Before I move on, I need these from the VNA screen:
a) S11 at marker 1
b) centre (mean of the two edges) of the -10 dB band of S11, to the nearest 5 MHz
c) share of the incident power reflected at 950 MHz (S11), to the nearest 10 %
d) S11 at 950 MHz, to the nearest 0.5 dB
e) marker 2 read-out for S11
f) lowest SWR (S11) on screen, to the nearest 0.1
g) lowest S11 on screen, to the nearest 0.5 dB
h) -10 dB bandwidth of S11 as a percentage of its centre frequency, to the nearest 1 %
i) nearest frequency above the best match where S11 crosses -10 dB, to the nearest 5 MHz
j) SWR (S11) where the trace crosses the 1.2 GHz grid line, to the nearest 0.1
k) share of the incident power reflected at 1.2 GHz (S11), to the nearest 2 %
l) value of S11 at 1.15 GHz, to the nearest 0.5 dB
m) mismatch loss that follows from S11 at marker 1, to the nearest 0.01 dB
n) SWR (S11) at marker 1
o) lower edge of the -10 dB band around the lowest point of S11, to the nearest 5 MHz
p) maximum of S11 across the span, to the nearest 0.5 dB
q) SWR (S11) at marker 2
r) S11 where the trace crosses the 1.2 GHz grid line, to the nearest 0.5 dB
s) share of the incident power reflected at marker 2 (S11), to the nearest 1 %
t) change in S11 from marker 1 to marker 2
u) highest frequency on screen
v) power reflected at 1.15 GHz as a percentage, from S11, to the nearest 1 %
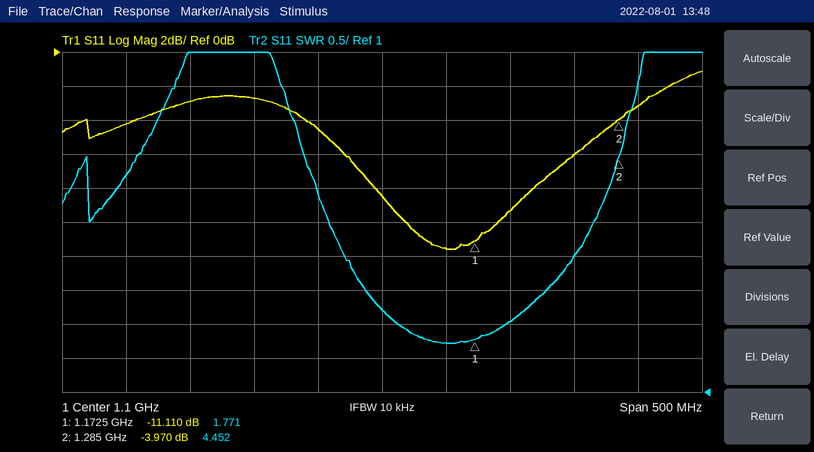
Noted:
-11.110 dB
1.155 GHz
50 %
-3.0 dB
-3.970 dB
1.7
-11.5 dB
6 %
1.190 GHz
2.0
12 %
-11.5 dB
0.35 dB
1.771
1.120 GHz
-1.0 dB
4.452
-9.5 dB
40 %
7.140 dB
1.35 GHz
7 %
